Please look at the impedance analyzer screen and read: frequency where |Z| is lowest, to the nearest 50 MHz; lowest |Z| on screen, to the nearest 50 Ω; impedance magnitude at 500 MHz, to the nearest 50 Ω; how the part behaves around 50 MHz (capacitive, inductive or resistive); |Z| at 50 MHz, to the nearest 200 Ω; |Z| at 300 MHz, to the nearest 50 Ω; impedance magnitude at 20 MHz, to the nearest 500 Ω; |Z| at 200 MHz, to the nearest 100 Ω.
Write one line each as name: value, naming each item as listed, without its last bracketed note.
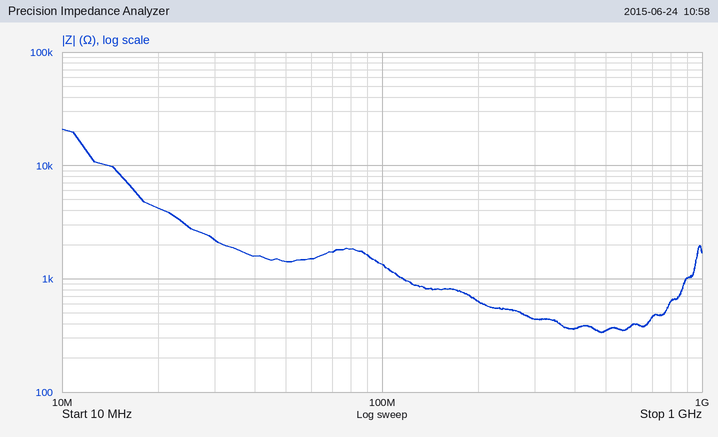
frequency where |Z| is lowest, to the nearest 50 MHz: 500 MHz
lowest |Z| on screen, to the nearest 50 Ω: 350 Ω
impedance magnitude at 500 MHz, to the nearest 50 Ω: 350 Ω
how the part behaves around 50 MHz: resistive
|Z| at 50 MHz, to the nearest 200 Ω: 1.4 kΩ
|Z| at 300 MHz, to the nearest 50 Ω: 450 Ω
impedance magnitude at 20 MHz, to the nearest 500 Ω: 4.0 kΩ
|Z| at 200 MHz, to the nearest 100 Ω: 600 Ω
